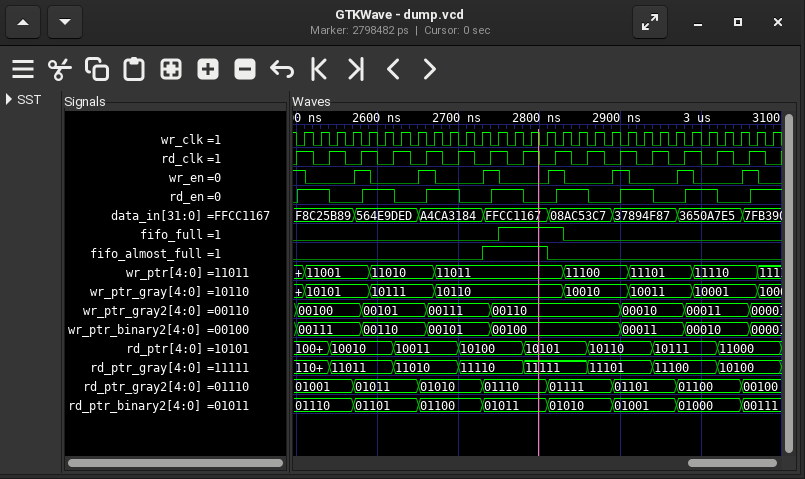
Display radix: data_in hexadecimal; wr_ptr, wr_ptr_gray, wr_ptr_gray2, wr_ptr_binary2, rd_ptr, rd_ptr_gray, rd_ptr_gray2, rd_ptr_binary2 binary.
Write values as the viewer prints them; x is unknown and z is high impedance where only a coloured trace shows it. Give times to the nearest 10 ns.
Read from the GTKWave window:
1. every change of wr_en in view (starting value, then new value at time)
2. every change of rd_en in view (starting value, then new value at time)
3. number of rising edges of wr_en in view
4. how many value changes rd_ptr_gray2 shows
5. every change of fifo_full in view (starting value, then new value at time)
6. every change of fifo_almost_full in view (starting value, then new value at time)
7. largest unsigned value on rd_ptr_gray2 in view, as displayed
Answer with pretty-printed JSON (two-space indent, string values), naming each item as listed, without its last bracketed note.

{
  "every change of wr_en in view": "1, 0 at 2510 ns, 1 at 2570 ns, 0 at 2590 ns, 1 at 2650 ns, 0 at 2670 ns, 1 at 2730 ns, 0 at 2750 ns, 1 at 2810 ns, 0 at 2830 ns, 1 at 2890 ns, 0 at 2910 ns, 1 at 2970 ns, 0 at 2990 ns, 1 at 3050 ns, 0 at 3070 ns",
  "every change of rd_en in view": "0, 1 at 2500 ns, 0 at 2540 ns, 1 at 2580 ns, 0 at 2620 ns, 1 at 2660 ns, 0 at 2700 ns, 1 at 2740 ns, 0 at 2780 ns, 1 at 2820 ns, 0 at 2860 ns, 1 at 2900 ns, 0 at 2940 ns, 1 at 2980 ns, 0 at 3020 ns, 1 at 3060 ns",
  "number of rising edges of wr_en in view": "7",
  "how many value changes rd_ptr_gray2 shows": "7",
  "every change of fifo_full in view": "0, 1 at 2750 ns, 0 at 2830 ns",
  "every change of fifo_almost_full in view": "0, 1 at 2730 ns, 0 at 2810 ns",
  "largest unsigned value on rd_ptr_gray2 in view, as displayed": "01111"
}
